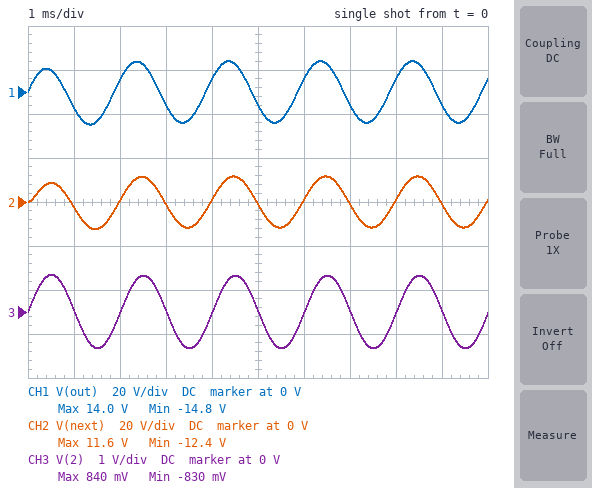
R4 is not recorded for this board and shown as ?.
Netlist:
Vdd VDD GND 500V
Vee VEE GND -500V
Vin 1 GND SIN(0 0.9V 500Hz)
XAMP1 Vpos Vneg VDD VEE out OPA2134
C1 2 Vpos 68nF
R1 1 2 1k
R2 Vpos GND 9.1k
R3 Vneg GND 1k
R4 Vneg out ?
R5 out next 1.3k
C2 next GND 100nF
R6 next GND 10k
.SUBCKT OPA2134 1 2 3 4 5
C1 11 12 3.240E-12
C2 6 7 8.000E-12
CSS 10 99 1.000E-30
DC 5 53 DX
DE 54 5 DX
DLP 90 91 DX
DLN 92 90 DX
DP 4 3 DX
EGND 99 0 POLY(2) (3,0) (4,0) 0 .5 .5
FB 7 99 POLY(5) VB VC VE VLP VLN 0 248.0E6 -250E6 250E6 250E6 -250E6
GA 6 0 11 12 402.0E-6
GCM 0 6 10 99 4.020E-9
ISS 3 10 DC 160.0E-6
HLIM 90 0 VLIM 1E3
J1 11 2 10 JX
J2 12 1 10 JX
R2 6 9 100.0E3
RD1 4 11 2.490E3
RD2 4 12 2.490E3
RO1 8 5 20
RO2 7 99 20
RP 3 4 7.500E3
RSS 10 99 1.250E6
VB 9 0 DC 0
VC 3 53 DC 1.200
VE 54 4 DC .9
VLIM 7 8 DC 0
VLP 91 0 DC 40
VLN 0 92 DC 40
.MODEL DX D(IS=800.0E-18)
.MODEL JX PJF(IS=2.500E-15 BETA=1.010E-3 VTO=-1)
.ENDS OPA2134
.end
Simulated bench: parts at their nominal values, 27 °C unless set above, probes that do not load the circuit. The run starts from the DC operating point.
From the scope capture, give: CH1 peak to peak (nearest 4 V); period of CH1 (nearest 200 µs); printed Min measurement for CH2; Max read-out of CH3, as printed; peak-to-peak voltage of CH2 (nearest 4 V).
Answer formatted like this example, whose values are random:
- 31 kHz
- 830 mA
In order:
- 28 V
- 2.0 ms
- -12.4 V
- 840 mV
- 24 V
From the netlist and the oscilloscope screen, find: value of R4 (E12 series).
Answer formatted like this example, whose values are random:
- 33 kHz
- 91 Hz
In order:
- 18 kΩ
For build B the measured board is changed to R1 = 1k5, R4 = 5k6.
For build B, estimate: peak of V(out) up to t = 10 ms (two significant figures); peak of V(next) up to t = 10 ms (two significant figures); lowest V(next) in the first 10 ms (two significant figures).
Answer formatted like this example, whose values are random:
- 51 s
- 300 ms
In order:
- 4.7 V
- 3.9 V
- -4.1 V
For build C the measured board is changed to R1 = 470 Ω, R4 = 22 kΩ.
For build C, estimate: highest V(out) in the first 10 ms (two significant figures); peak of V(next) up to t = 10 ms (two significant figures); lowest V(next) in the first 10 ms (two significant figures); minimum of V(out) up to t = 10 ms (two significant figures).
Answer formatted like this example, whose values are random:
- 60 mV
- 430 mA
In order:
- 18 V
- 15 V
- -16 V
- -19 V
